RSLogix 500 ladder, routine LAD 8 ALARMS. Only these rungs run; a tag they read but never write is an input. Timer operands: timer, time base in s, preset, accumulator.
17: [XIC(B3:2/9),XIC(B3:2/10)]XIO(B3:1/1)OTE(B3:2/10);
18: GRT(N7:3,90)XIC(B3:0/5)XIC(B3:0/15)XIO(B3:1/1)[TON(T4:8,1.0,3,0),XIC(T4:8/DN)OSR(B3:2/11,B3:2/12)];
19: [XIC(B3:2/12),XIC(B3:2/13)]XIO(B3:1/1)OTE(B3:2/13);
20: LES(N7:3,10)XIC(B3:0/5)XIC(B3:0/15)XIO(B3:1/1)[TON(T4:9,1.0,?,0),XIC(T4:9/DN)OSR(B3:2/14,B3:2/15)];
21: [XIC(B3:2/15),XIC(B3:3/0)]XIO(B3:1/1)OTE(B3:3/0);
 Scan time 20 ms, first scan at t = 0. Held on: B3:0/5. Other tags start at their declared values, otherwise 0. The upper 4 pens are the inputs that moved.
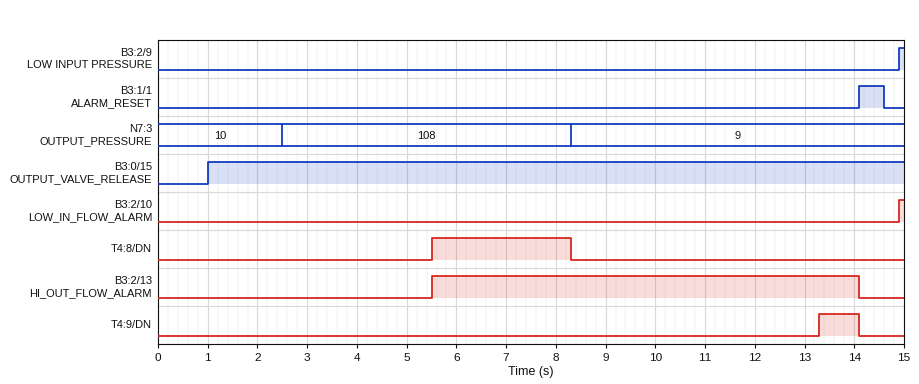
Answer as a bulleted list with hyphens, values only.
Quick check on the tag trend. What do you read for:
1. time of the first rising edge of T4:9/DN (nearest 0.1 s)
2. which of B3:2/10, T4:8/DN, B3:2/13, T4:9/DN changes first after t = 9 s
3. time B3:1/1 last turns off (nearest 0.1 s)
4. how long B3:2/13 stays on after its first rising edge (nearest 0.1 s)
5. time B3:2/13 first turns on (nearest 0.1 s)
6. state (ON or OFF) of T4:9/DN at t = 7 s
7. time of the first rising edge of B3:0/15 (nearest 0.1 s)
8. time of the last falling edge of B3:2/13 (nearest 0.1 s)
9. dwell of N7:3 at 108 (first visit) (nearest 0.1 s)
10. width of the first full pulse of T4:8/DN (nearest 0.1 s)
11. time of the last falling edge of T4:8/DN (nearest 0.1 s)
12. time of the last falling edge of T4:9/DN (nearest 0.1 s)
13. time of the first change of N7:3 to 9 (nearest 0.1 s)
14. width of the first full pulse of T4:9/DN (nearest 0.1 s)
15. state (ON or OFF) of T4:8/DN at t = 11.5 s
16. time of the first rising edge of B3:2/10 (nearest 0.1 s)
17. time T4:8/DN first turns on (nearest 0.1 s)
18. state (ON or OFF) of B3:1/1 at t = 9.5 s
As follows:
- 13.3 s
- T4:9/DN
- 14.6 s
- 8.6 s
- 5.5 s
- OFF
- 1.0 s
- 14.1 s
- 5.8 s
- 2.8 s
- 8.3 s
- 14.1 s
- 8.3 s
- 0.8 s
- OFF
- 14.9 s
- 5.5 s
- OFF
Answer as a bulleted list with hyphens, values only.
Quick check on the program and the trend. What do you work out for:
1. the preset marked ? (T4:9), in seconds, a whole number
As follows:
- 5 s
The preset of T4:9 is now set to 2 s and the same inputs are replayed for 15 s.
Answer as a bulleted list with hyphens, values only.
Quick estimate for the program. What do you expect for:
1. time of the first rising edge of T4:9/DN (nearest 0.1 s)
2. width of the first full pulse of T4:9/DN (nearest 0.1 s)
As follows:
- 10.3 s
- 3.8 s
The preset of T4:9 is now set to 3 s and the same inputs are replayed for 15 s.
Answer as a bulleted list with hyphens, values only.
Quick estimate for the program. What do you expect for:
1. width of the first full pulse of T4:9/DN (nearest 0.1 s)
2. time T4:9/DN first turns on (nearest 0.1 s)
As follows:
- 2.8 s
- 11.3 s
